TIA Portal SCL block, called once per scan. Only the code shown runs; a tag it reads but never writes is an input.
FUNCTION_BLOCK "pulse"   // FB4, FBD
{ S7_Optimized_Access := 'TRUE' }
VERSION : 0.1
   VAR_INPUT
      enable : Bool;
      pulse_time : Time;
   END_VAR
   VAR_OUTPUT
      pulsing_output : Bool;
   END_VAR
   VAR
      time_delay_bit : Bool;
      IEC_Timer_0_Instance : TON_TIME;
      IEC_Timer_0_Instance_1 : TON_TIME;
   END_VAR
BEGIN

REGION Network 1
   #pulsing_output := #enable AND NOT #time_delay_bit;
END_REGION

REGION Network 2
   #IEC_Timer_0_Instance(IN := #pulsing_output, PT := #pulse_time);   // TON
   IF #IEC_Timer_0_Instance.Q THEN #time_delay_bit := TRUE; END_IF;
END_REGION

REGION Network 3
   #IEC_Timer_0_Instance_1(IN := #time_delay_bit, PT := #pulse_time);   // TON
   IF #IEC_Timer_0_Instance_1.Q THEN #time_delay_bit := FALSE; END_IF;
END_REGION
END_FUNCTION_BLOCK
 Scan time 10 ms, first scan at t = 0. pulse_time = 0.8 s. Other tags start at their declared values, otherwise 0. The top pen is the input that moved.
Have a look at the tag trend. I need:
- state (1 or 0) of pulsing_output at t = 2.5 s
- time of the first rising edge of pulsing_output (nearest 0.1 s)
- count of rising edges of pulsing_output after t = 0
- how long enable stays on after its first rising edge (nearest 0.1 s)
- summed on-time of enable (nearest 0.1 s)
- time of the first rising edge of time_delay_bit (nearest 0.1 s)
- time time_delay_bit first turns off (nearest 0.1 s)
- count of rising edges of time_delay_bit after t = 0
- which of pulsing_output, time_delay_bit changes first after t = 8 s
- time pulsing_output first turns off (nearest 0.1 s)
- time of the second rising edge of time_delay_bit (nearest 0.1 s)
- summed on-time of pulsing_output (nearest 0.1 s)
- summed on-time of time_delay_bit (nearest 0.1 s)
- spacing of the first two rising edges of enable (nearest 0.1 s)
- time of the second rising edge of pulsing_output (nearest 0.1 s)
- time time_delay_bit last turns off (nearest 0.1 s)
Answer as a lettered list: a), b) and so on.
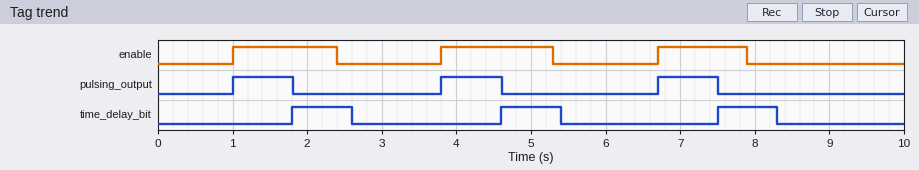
a) 0
b) 1.0 s
c) 3
d) 1.4 s
e) 4.1 s
f) 1.8 s
g) 2.6 s
h) 3
i) time_delay_bit
j) 1.8 s
k) 4.6 s
l) 2.4 s
m) 2.4 s
n) 2.8 s
o) 3.8 s
p) 8.3 s
